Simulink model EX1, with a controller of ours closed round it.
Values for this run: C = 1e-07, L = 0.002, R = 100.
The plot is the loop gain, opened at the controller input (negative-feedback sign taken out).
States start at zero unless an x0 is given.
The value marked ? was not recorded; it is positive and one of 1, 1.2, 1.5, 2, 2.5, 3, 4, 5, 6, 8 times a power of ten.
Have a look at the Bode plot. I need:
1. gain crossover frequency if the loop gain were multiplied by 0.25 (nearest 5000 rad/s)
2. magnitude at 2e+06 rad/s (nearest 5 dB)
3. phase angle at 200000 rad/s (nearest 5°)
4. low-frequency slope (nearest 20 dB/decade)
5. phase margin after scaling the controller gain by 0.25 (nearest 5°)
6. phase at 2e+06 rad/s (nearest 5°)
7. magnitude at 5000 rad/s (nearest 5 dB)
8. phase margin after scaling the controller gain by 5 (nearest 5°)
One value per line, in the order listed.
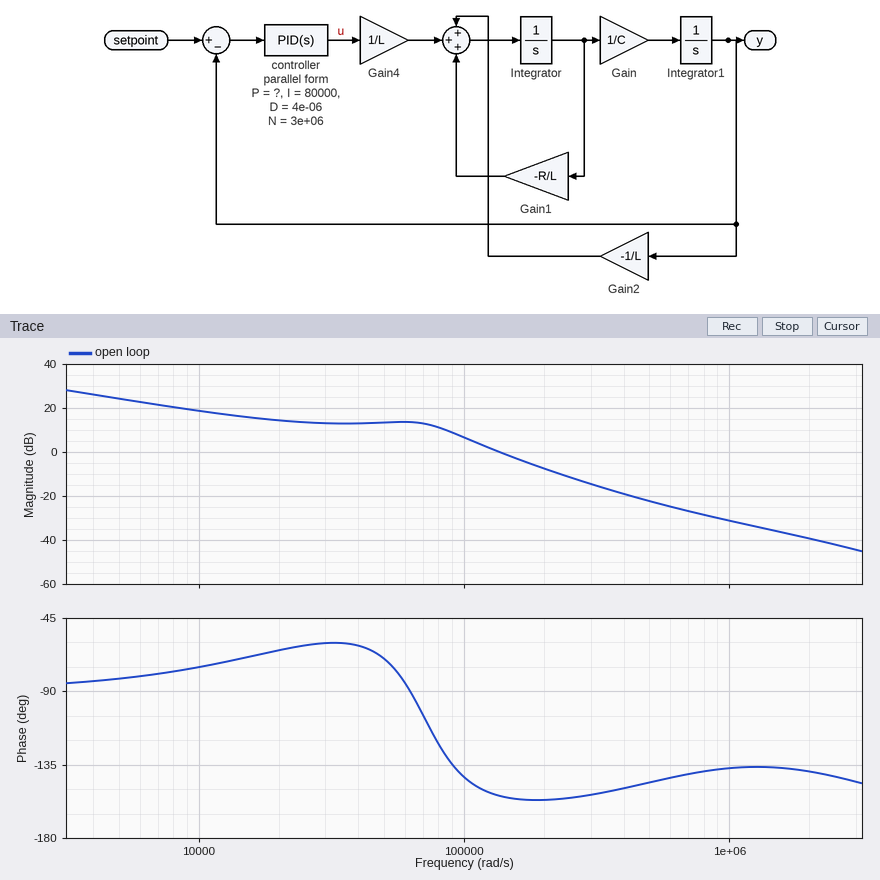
75000 rad/s
-40 dB
-155°
-20 dB/decade
65°
-140°
25 dB
25°
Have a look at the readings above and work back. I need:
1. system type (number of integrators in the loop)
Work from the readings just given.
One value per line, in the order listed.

1
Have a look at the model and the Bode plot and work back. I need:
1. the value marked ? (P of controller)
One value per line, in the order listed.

3
